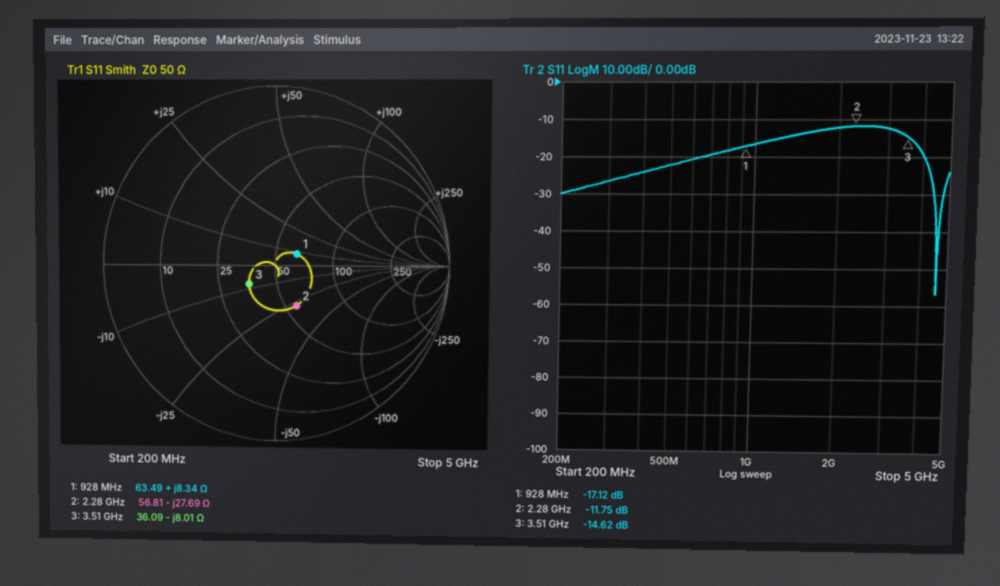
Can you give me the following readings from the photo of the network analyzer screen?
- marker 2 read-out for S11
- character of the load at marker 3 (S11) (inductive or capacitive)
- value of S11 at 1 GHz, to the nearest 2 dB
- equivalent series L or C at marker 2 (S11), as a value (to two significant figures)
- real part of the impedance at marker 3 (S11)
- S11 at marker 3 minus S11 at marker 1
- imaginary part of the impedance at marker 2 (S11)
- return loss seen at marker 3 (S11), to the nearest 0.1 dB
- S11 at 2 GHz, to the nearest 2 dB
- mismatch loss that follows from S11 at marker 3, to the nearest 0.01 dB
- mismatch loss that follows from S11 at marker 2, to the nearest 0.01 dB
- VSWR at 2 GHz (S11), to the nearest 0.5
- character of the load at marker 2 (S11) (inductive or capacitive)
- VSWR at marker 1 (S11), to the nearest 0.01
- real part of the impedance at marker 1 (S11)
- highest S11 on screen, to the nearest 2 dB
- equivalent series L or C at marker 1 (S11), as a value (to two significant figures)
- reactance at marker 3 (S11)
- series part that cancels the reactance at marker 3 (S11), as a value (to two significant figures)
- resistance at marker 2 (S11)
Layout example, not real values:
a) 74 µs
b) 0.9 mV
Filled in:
a) -11.75 dB
b) capacitive
c) -16 dB
d) 2.5 pF
e) 36.09 Ω
f) 2.50 dB
g) -27.69 Ω
h) 14.6 dB
i) -12 dB
j) 0.15 dB
k) 0.30 dB
l) 1.5
m) capacitive
n) 1.32
o) 63.49 Ω
p) -12 dB
q) 1.4 nH
r) -8.01 Ω
s) 360 pH
t) 56.81 Ω
